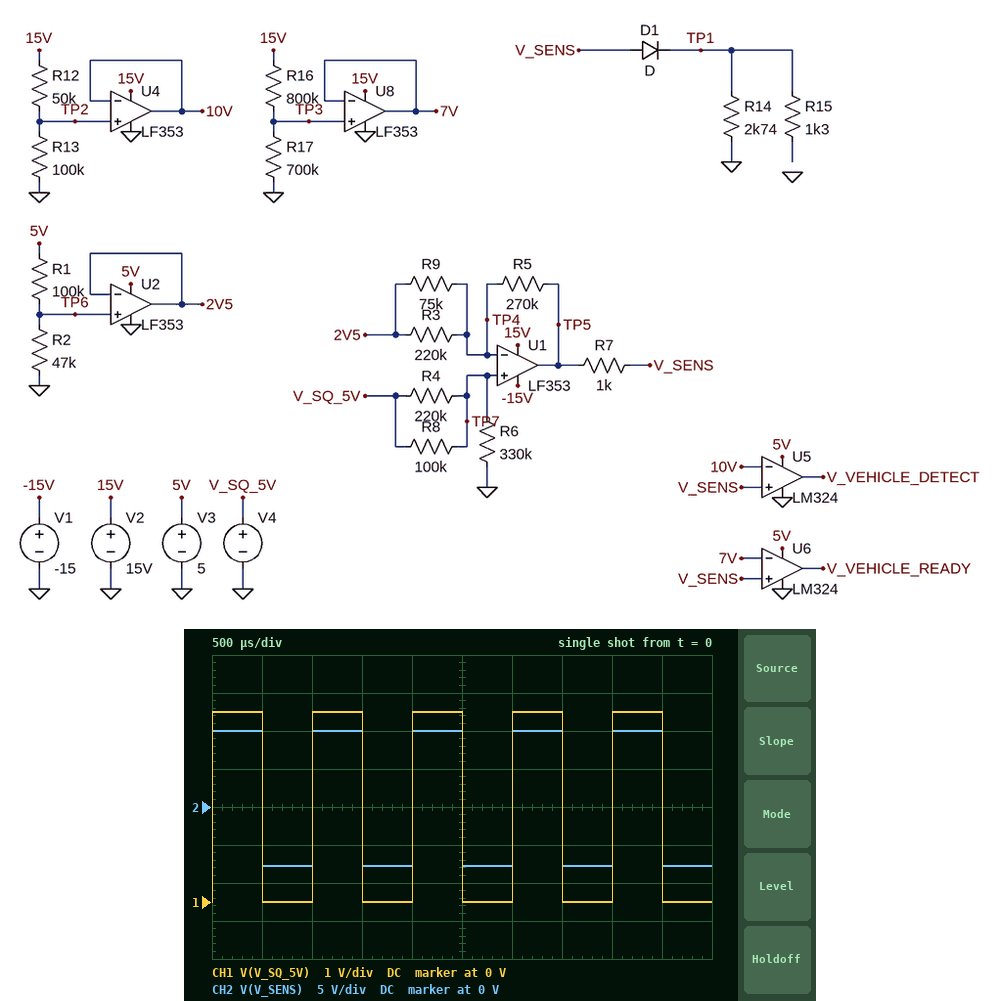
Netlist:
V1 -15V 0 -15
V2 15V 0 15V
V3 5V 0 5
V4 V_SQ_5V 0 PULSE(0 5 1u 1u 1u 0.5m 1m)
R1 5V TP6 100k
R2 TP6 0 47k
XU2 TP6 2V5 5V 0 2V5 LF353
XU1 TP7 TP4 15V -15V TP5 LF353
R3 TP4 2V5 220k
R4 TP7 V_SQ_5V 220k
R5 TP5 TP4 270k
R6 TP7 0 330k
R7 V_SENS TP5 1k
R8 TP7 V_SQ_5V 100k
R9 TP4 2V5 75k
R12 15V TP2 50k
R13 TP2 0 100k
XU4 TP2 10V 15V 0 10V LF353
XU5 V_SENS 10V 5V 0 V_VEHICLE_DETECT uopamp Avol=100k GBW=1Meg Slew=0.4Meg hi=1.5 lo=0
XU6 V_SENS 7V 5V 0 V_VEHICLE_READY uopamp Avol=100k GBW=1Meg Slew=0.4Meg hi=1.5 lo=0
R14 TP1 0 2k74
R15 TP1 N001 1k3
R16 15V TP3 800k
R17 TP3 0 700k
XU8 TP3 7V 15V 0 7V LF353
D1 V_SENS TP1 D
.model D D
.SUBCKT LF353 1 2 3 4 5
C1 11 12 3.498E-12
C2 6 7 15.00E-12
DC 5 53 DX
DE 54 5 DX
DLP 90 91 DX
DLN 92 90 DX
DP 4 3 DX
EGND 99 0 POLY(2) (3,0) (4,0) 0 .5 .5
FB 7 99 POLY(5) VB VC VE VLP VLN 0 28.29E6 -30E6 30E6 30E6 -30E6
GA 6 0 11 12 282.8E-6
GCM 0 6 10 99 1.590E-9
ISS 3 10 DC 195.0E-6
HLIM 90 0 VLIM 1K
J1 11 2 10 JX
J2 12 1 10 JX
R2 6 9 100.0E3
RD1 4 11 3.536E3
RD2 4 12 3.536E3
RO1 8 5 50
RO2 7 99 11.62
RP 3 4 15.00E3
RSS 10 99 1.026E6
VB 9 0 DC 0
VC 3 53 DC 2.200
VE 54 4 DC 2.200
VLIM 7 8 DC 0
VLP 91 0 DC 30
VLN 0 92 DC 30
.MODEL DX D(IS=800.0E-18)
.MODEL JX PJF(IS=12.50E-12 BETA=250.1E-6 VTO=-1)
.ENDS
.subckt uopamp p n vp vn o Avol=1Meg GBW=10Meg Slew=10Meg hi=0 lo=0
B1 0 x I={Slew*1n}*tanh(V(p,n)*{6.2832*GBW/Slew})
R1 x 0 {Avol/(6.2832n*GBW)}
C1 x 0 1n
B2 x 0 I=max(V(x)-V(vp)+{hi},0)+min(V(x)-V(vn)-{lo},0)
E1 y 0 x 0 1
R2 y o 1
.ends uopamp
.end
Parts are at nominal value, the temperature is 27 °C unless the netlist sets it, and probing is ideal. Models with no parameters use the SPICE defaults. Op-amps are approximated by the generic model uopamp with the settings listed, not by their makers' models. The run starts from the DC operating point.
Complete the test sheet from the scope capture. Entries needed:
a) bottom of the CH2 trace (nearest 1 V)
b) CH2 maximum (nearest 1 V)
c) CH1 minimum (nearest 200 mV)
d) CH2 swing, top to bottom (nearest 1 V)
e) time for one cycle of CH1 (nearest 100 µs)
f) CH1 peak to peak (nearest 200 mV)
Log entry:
-8 V
10 V
0 V
18 V
1.0 ms
5.0 V
